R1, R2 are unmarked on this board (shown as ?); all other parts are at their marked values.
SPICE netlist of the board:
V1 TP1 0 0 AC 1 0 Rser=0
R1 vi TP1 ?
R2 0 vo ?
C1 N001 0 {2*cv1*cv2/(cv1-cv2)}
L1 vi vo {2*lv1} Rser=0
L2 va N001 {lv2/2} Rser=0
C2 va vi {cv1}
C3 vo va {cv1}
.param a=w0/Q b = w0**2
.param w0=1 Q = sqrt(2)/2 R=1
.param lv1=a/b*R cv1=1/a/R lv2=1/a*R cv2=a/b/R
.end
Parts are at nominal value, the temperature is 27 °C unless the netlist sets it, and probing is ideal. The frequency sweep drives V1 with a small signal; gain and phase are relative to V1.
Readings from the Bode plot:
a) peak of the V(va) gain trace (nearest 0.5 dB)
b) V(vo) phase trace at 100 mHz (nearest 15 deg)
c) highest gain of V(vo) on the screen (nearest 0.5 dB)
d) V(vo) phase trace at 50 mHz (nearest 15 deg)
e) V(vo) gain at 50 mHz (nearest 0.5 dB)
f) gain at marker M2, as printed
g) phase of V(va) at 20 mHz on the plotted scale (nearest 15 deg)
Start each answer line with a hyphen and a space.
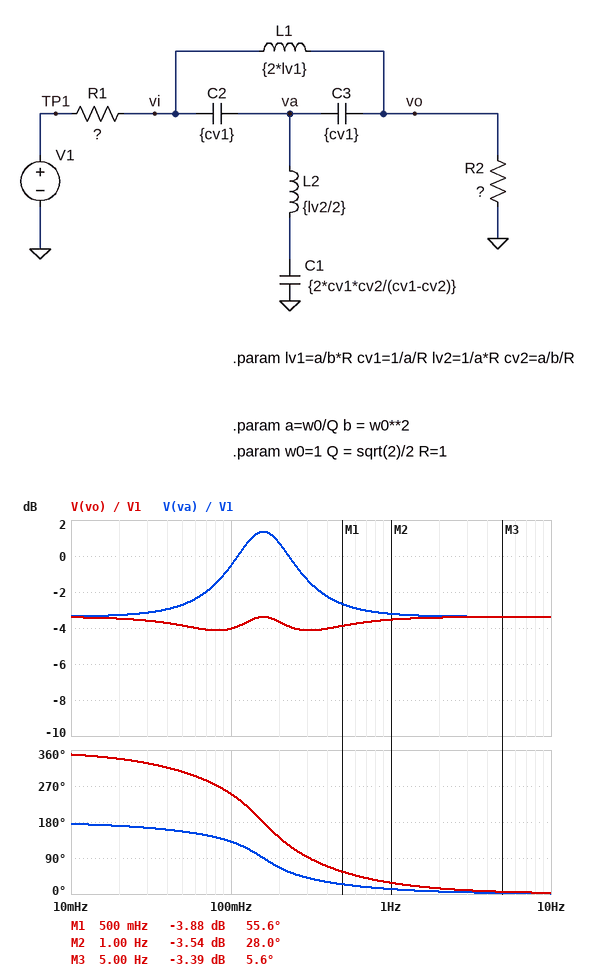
- 1.5 dB
- 255 deg
- -3.5 dB
- 300 deg
- -4.0 dB
- -3.54 dB
- 165 deg
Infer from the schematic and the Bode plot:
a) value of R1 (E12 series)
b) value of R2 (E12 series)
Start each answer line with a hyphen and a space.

- 0.39 Ω
- 0.82 Ω
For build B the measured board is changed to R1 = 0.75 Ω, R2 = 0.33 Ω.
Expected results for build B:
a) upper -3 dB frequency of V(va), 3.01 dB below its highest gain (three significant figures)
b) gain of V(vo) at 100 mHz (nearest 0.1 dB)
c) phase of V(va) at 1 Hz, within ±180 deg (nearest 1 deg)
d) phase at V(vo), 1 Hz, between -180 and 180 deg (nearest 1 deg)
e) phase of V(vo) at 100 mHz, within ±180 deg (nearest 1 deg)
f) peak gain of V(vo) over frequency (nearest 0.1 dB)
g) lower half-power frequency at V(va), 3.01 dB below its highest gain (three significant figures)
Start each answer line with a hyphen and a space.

- 246 mHz
- -11.4 dB
- -6 deg
- 29 deg
- -109 deg
- -10.3 dB
- 103 mHz
